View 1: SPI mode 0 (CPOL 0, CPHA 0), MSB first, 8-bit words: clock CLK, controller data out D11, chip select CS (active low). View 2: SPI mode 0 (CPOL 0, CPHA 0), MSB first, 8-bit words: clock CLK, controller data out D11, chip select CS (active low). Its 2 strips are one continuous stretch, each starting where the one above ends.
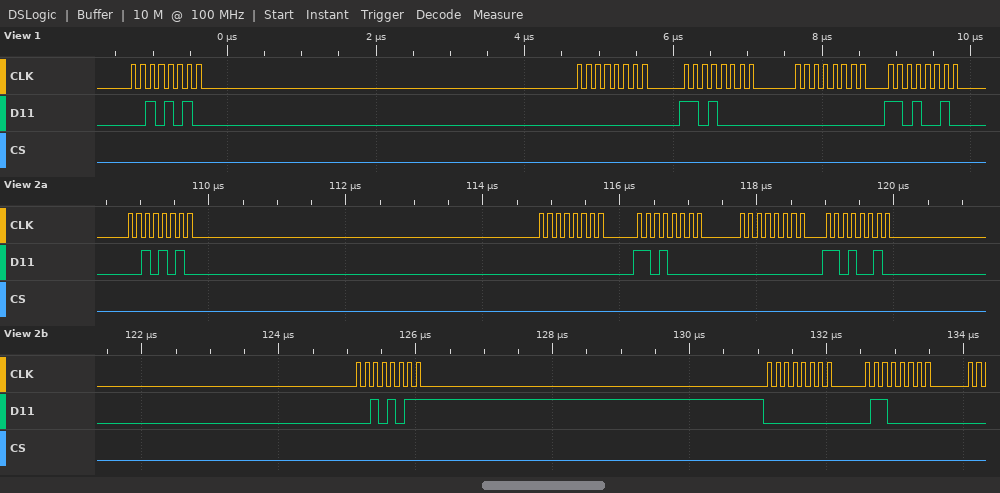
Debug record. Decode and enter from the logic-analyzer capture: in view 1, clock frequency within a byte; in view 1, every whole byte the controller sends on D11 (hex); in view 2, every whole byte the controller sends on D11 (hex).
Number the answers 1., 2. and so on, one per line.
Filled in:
1. 8 MHz
2. 2A 00 D0 00 D2
3. 2A 00 D0 00 D2 2B 00 60
